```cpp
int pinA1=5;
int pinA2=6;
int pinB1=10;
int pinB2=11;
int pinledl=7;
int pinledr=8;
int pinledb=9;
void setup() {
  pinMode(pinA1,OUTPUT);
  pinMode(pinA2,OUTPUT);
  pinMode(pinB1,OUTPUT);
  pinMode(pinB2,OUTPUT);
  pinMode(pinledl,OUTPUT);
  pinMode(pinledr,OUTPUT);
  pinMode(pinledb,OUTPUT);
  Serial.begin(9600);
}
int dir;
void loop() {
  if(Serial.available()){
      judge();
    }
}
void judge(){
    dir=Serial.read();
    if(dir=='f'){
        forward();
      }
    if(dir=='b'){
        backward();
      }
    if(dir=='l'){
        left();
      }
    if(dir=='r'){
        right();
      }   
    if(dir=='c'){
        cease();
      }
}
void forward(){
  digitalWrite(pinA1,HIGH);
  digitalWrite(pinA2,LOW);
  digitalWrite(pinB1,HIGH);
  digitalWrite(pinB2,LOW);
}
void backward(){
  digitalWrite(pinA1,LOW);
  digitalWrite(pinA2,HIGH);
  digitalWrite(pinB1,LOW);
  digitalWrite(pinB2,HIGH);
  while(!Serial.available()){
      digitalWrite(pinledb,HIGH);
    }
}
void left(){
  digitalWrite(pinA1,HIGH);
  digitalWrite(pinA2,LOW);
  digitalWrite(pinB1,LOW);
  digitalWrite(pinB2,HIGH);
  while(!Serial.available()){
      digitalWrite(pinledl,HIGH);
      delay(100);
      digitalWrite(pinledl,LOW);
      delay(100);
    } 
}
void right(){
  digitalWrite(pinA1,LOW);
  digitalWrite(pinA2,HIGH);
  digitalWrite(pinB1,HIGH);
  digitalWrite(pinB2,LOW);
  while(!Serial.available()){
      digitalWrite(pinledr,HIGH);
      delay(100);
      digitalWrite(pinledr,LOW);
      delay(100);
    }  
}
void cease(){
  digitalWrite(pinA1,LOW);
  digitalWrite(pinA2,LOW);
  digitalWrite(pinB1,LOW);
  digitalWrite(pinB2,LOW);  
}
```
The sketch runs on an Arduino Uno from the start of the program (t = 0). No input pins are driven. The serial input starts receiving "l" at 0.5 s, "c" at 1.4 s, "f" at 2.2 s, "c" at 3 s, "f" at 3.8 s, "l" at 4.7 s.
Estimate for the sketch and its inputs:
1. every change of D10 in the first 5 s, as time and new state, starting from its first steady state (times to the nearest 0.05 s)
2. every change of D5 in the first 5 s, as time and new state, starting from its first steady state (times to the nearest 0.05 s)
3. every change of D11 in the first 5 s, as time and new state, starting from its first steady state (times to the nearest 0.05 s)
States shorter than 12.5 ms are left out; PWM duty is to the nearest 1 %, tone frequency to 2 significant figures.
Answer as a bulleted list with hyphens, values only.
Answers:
- 0 s low; 2.2 s high; 3 s low; 3.8 s high; 4.7 s low
- 0 s low; 0.5 s high; 1.5 s low; 2.2 s high; 3 s low; 3.8 s high
- 0 s low; 0.5 s high; 1.5 s low; 4.7 s high
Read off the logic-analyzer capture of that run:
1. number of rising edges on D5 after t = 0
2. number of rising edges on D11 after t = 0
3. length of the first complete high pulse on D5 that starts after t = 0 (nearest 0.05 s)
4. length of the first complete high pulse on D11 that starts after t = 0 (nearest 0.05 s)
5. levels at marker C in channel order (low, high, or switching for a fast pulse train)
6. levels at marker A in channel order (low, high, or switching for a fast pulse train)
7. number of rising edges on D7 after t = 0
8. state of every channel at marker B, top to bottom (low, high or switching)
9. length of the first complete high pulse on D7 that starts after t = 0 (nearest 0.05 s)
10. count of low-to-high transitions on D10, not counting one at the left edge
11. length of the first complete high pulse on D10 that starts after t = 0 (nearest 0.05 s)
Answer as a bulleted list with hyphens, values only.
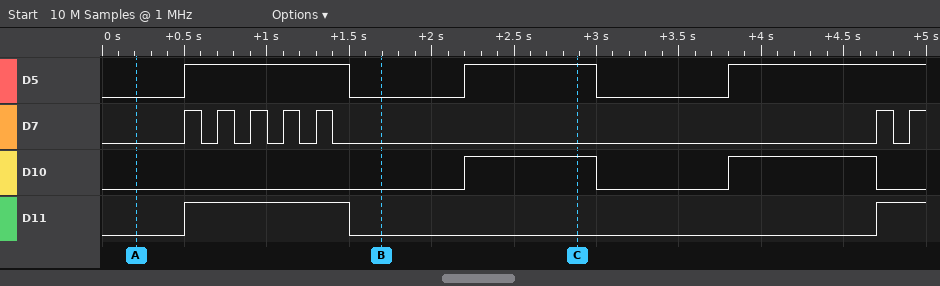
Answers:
- 3
- 2
- 1.00 s
- 1.00 s
- D5 high, D7 low, D10 high, D11 low
- D5 low, D7 low, D10 low, D11 low
- 7
- D5 low, D7 low, D10 low, D11 low
- 0.10 s
- 2
- 0.80 s
